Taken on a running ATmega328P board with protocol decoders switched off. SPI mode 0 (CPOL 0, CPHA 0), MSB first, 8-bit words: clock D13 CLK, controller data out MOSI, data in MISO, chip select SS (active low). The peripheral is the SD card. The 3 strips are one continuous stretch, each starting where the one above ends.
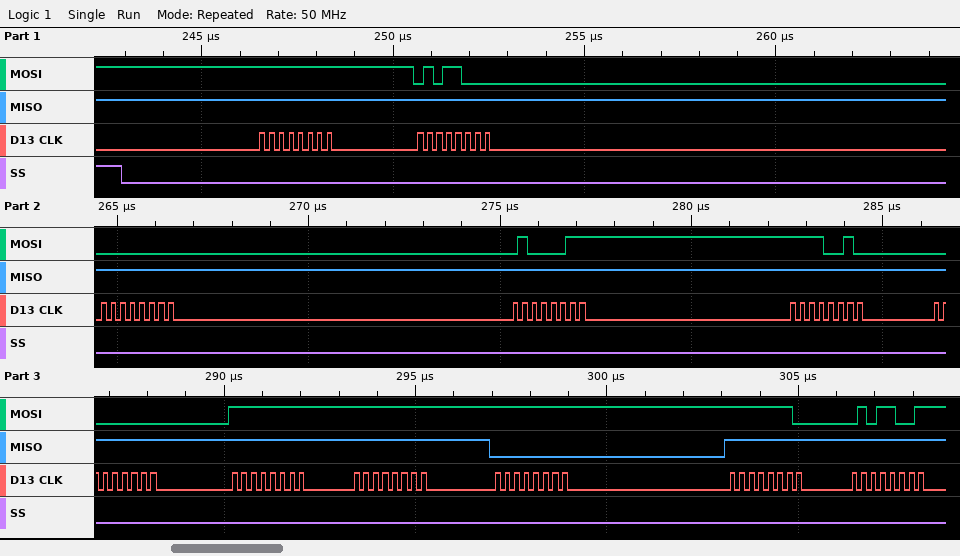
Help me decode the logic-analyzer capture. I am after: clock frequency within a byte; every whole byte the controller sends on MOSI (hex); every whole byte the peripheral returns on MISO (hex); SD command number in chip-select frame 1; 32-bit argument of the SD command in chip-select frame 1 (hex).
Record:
4 MHz
FF 58 00 43 F2 00 FF FF FF FE 59
FF FF FF FF FF FF FF FF 00 FF FF
CMD24
0x0043F200
